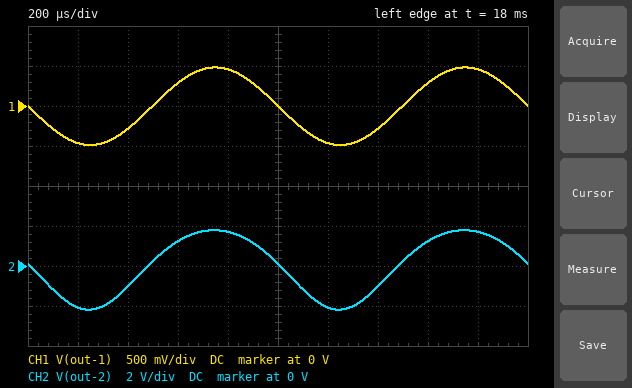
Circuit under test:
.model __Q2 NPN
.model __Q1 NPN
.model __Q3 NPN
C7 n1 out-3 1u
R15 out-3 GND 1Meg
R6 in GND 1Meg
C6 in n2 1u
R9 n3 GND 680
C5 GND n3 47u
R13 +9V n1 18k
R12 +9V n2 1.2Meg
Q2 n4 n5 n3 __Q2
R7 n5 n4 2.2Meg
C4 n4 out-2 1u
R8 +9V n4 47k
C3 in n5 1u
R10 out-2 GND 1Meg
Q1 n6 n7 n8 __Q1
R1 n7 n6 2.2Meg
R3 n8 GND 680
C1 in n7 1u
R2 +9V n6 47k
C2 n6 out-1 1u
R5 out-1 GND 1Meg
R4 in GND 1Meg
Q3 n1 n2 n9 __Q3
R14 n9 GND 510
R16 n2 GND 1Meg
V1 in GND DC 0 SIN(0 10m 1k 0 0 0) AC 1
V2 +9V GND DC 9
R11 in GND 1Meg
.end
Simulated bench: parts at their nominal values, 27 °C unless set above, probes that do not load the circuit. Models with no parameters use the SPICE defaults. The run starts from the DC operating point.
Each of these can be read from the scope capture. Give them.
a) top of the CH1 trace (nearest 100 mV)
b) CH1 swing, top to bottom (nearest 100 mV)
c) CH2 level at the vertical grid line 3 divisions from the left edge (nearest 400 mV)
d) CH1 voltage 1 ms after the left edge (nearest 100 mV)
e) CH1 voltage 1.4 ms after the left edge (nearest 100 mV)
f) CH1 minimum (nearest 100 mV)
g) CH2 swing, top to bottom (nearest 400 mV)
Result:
500 mV
1.0 V
1.2 V
0 V
-300 mV
-500 mV
4.0 V
